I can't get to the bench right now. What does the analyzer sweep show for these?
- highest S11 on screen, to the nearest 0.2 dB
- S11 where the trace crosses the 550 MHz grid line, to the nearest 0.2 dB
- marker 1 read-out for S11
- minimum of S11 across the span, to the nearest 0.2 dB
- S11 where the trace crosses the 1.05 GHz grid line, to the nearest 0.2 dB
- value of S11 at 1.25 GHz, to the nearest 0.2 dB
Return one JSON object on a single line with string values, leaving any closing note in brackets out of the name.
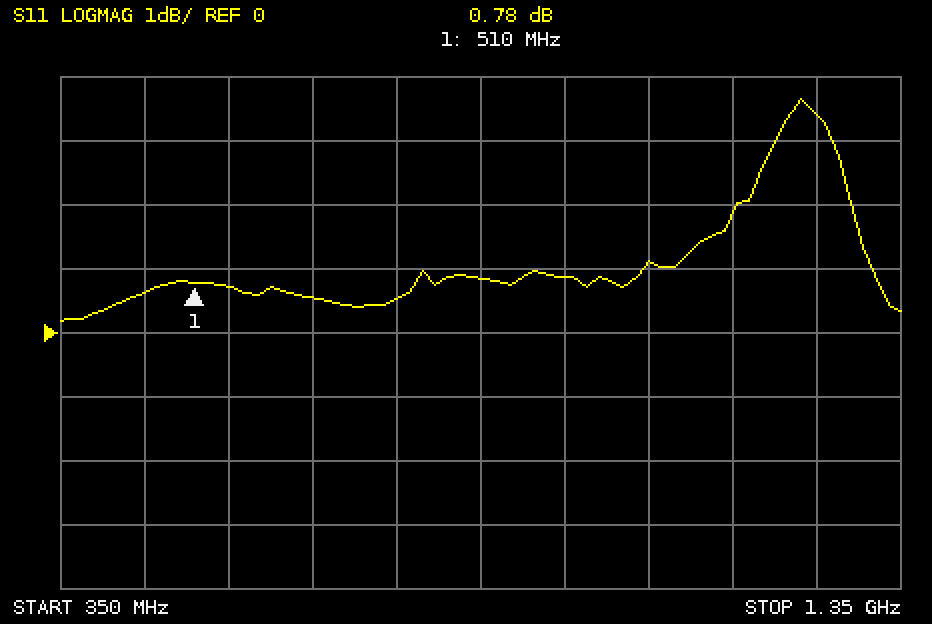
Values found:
{"highest S11 on screen, to the nearest 0.2 dB": "3.6 dB", "S11 where the trace crosses the 550 MHz grid line, to the nearest 0.2 dB": "0.8 dB", "marker 1 read-out for S11": "0.78 dB", "minimum of S11 across the span, to the nearest 0.2 dB": "0.2 dB", "S11 where the trace crosses the 1.05 GHz grid line, to the nearest 0.2 dB": "1.2 dB", "value of S11 at 1.25 GHz, to the nearest 0.2 dB": "3.4 dB"}
